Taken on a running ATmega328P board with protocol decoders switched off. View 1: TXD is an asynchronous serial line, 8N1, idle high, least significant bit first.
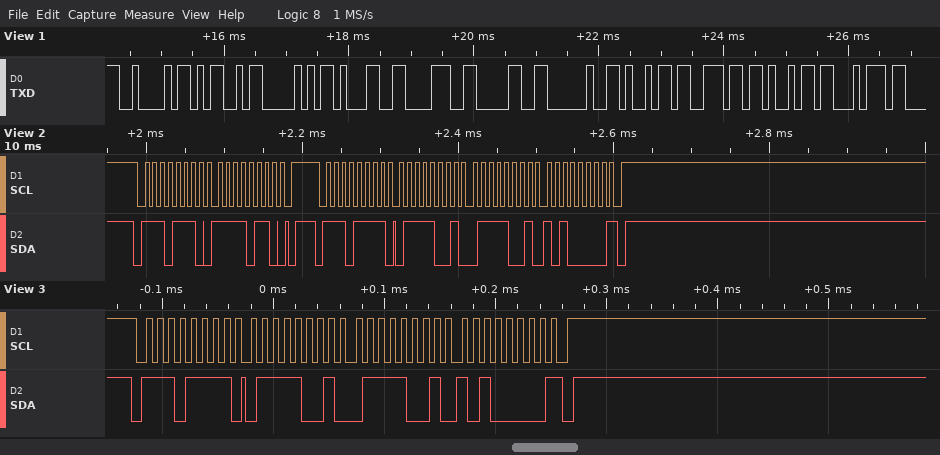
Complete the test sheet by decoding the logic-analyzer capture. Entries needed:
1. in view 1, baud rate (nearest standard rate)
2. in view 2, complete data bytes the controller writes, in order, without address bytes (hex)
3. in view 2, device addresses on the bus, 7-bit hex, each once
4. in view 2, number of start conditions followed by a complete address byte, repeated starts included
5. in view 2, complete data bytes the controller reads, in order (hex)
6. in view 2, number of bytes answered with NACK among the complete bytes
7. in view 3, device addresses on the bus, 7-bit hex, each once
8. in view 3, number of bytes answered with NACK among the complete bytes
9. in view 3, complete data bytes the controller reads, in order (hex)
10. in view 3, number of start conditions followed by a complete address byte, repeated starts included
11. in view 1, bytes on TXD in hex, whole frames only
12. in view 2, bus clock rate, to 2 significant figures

9600 baud
F6
0x77
2
79 79 A0
1
0x77
1
79 79 A0
1
42 4D 50 31 38 30 20 69 6E 69 74
100 kHz
